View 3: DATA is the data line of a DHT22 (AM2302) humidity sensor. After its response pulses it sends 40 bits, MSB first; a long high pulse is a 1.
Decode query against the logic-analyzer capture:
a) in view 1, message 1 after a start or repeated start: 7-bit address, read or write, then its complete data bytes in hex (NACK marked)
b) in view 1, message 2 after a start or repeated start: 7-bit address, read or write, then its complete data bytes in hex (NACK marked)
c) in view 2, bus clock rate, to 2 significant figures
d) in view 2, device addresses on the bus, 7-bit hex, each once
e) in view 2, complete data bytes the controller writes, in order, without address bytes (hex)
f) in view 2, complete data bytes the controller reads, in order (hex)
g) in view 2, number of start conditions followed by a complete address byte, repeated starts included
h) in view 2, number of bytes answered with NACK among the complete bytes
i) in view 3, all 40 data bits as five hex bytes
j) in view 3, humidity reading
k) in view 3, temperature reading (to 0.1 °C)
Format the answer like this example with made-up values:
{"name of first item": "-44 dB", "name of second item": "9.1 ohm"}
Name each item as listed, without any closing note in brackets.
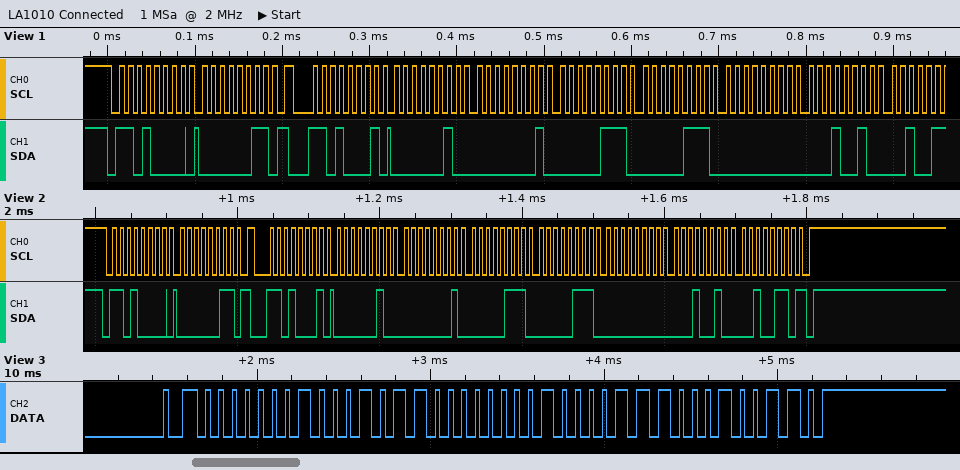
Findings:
{"in view 1, message 1 after a start or repeated start: 7-bit address, read or write, then its complete data bytes in hex": "0x68 write: 03", "in view 1, message 2 after a start or repeated start: 7-bit address, read or write, then its complete data bytes in hex": "0x68 read: 02 01 07 07 00 12", "in view 2, bus clock rate, to 2 significant figures": "100 kHz", "in view 2, device addresses on the bus, 7-bit hex, each once": "0x68", "in view 2, complete data bytes the controller writes, in order, without address bytes": "03", "in view 2, complete data bytes the controller reads, in order": "02 01 07 07 00 12 26", "in view 2, number of start conditions followed by a complete address byte, repeated starts included": "2", "in view 2, number of bytes answered with NACK among the complete bytes": "1", "in view 3, all 40 data bits as five hex bytes": "01 16 01 0E 26", "in view 3, humidity reading": "27.8 %", "in view 3, temperature reading": "27.0 °C"}
